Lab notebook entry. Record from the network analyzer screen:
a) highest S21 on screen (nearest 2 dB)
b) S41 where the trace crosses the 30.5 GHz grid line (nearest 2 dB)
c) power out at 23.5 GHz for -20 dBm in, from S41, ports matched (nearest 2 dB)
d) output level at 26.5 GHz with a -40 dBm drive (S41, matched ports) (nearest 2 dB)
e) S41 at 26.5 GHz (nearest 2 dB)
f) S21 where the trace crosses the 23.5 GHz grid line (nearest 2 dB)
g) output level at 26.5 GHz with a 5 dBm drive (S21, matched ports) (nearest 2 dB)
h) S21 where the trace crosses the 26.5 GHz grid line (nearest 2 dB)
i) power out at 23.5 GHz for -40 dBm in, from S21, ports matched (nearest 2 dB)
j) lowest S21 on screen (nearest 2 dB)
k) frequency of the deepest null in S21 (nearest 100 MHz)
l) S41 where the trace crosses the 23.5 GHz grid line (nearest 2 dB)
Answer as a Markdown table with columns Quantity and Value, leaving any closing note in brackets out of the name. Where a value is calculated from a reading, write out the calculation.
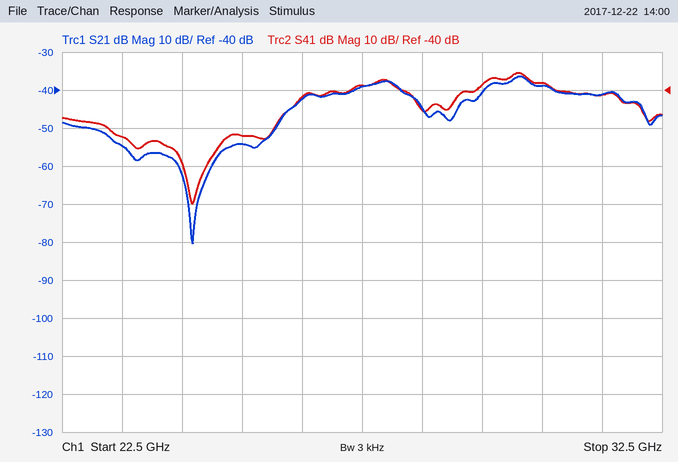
| Quantity | Value |
|---|---|
| highest S21 on screen | -36 dB |
| S41 where the trace crosses the 30.5 GHz grid line | -38 dB |
| power out at 23.5 GHz for -20 dBm in, from S41, ports matched | -20 dBm + (-52 dB) = -72 dBm |
| output level at 26.5 GHz with a -40 dBm drive (S41, matched ports) | -40 dBm + (-42 dB) = -82 dBm |
| S41 at 26.5 GHz | -42 dB |
| S21 where the trace crosses the 23.5 GHz grid line | -54 dB |
| output level at 26.5 GHz with a 5 dBm drive (S21, matched ports) | 5 dBm + (-42 dB) = -38 dBm |
| S21 where the trace crosses the 26.5 GHz grid line | -42 dB |
| power out at 23.5 GHz for -40 dBm in, from S21, ports matched | -40 dBm + (-54 dB) = -94 dBm |
| lowest S21 on screen | -80 dB |
| frequency of the deepest null in S21 | 24.7 GHz |
| S41 where the trace crosses the 23.5 GHz grid line | -52 dB |
